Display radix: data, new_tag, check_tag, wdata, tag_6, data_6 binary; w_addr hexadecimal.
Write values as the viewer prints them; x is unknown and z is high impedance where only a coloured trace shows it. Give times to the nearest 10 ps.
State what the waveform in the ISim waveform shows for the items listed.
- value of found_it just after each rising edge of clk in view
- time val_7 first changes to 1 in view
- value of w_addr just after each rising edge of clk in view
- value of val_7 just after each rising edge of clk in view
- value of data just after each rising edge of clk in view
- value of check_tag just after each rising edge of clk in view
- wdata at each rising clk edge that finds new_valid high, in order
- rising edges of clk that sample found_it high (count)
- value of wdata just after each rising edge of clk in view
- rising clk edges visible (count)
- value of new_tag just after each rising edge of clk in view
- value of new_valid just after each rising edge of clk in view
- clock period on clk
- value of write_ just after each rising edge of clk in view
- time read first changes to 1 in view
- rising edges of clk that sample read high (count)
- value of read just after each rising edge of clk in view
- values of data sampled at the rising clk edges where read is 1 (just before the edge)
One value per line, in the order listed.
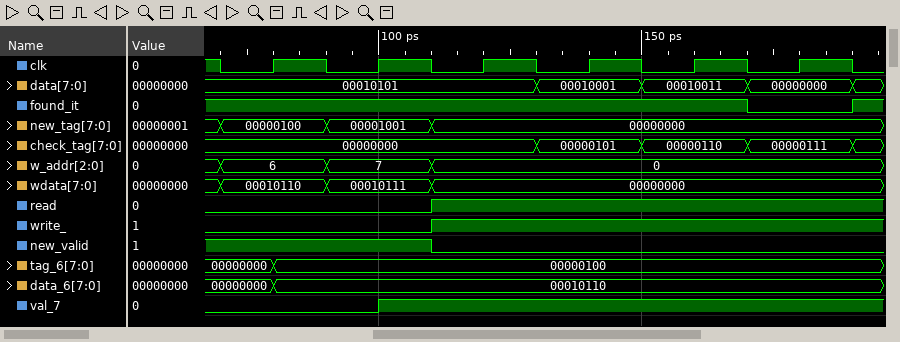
1 1 1 1 1 0
100 ps
6, 7, 0, 0, 0, 0
0 1 1 1 1 1
00010101, 00010101, 00010101, 00010001, 00010011, 00000000
00000000, 00000000, 00000000, 00000101, 00000110, 00000111
00010110, 00010111
5
00010110, 00010111, 00000000, 00000000, 00000000, 00000000
6
00000100, 00001001, 00000000, 00000000, 00000000, 00000000
1 1 0 0 0 0
20 ps
0 0 1 1 1 1
110 ps
4
0 0 1 1 1 1
00010101, 00010001, 00010011, 00000000
